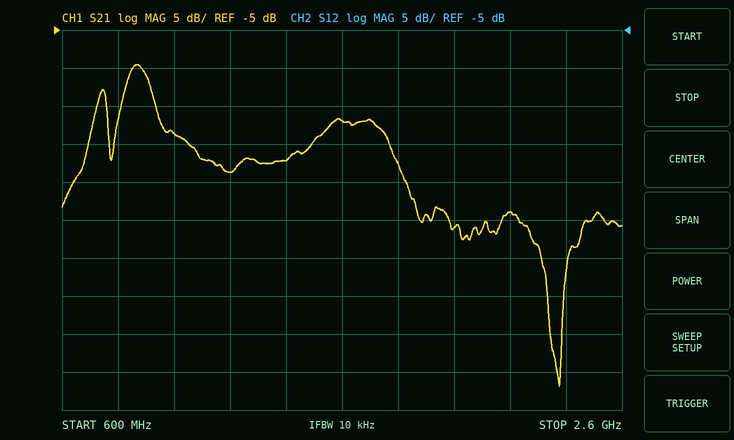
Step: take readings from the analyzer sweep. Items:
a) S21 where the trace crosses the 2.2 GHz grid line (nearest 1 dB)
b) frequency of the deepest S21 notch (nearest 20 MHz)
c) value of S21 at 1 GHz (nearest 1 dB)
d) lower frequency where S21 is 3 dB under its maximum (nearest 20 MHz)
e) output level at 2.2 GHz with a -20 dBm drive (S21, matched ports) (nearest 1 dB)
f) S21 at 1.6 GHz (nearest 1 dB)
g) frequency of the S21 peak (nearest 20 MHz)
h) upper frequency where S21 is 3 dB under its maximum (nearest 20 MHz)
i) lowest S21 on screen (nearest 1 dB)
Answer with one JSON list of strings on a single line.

["-29 dB", "2.38 GHz", "-19 dB", "820 MHz", "-49 dBm", "-17 dB", "860 MHz", "920 MHz", "-52 dB"]
